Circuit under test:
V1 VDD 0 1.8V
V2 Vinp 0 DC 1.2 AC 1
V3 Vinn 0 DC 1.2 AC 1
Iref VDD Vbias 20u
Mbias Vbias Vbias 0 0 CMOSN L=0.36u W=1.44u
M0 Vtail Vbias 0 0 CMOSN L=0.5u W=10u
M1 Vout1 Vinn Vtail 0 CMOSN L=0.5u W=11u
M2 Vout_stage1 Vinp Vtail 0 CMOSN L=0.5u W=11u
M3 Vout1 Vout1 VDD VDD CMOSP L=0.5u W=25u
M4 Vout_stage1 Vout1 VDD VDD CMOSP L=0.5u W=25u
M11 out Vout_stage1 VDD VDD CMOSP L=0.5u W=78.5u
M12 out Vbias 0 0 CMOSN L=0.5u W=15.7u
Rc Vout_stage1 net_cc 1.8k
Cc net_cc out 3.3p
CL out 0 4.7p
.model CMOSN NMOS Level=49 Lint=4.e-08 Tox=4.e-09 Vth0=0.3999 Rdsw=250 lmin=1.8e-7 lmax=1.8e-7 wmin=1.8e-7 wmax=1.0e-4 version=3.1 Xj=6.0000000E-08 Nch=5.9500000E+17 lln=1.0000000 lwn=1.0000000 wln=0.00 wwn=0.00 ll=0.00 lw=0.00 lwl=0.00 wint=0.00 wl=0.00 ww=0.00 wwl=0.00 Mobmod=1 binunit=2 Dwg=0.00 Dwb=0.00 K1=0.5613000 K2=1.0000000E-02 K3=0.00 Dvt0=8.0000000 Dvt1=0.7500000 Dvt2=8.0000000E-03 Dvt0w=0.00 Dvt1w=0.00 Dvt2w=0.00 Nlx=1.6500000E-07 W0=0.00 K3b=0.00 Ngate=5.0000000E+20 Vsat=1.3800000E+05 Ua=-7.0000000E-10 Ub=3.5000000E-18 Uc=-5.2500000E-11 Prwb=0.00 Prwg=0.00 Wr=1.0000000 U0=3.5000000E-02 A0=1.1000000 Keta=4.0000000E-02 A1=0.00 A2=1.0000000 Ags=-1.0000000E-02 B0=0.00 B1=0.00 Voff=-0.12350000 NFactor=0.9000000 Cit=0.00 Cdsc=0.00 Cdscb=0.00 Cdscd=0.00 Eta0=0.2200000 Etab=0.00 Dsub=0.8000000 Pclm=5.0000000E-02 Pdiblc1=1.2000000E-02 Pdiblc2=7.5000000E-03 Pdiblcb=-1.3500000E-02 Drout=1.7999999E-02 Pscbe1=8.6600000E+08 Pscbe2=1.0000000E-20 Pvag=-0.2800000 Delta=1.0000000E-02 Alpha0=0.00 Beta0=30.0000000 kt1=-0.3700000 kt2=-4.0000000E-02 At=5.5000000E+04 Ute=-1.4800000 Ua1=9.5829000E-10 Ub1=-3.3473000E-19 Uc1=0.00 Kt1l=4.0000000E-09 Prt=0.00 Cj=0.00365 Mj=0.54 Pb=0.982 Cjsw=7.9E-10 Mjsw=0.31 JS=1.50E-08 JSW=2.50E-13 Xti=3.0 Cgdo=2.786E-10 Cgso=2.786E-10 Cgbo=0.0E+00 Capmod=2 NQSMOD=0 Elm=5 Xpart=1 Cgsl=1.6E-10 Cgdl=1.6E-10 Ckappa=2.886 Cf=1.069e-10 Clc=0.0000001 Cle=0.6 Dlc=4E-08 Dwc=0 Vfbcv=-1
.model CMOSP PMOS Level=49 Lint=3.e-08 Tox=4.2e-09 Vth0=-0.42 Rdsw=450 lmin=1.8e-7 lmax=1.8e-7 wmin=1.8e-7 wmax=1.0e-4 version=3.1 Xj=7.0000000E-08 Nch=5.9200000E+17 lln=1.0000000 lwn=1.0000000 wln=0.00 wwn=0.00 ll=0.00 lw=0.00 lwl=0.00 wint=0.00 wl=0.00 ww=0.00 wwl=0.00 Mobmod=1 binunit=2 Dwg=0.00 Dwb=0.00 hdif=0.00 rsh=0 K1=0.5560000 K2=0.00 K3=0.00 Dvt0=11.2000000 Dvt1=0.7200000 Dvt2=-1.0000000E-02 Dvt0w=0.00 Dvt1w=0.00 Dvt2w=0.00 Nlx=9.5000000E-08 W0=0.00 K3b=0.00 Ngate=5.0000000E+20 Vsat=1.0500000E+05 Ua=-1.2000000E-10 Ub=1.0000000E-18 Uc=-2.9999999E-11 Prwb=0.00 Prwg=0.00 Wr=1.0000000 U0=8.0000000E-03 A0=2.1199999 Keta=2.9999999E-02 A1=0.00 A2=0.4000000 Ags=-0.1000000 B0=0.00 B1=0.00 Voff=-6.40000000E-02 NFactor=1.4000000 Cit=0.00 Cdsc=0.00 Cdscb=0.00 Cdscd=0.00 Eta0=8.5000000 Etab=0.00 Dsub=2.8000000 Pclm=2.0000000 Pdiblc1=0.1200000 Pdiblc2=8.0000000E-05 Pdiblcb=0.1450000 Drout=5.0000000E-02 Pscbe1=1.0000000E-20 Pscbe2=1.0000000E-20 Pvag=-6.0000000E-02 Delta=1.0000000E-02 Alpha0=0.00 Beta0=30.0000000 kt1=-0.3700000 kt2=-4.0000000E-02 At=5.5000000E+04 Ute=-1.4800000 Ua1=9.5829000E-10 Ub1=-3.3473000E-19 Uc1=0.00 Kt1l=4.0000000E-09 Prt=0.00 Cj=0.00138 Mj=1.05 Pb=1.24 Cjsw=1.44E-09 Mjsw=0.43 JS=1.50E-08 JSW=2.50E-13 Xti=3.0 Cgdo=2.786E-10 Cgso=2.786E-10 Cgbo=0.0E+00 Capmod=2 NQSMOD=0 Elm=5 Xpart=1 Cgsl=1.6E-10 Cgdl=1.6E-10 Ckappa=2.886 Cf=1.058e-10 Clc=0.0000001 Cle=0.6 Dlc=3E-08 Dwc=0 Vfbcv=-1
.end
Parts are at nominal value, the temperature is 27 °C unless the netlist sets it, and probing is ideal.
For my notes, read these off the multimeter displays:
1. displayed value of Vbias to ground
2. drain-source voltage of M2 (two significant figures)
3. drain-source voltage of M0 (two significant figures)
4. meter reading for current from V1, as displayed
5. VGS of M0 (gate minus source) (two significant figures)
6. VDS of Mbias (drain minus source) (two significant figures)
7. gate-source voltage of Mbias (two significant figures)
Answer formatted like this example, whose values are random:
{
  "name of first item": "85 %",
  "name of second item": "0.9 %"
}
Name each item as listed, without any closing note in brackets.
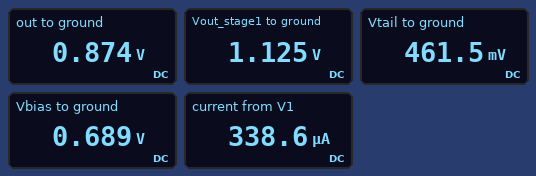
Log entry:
{
  "displayed value of Vbias to ground": "0.689 V",
  "drain-source voltage of M2": "660 mV",
  "drain-source voltage of M0": "460 mV",
  "meter reading for current from V1, as displayed": "338.6 µA",
  "VGS of M0 (gate minus source)": "690 mV",
  "VDS of Mbias (drain minus source)": "690 mV",
  "gate-source voltage of Mbias": "690 mV"
}
